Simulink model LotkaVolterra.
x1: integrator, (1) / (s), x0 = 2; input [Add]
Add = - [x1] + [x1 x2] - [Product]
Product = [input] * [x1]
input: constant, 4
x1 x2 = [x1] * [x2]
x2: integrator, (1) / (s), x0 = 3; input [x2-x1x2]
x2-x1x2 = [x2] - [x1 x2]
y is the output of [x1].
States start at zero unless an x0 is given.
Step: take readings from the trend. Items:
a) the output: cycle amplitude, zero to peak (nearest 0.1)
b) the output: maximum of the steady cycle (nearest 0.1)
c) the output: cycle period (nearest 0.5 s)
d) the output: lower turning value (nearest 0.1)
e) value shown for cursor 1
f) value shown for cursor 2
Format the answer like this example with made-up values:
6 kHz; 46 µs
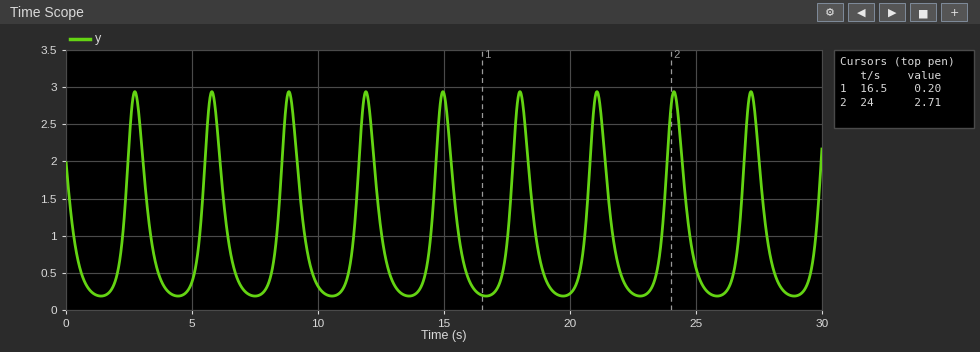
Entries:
1.4; 2.9; 3.0 s; 0.2; 0.20; 2.71
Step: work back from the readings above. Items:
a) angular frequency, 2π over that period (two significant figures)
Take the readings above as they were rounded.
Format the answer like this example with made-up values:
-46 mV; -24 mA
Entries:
2.1 rad/s
